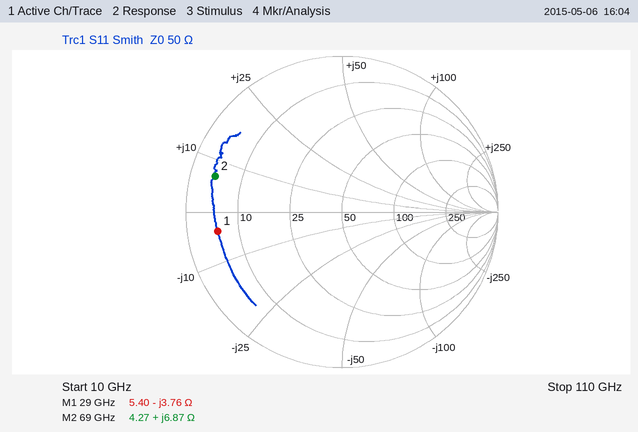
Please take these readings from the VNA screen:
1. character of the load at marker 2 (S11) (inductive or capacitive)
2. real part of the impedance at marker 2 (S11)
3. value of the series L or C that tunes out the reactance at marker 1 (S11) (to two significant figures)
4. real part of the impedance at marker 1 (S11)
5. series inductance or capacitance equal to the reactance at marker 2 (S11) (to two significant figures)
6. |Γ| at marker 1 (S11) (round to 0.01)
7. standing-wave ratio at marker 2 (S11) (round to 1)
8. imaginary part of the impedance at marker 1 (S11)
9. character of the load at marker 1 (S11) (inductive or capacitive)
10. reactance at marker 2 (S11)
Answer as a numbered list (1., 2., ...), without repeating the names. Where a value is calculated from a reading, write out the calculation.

1. inductive
2. 4.27 Ω
3. L = 3.76 Ω/(2π × 29 GHz) ≈ 21 pH
4. 5.40 Ω
5. L = 6.87 Ω/(2π × 69 GHz) ≈ 16 pH
6. 0.81
7. 12
8. -3.76 Ω
9. capacitive
10. +6.87 Ω
